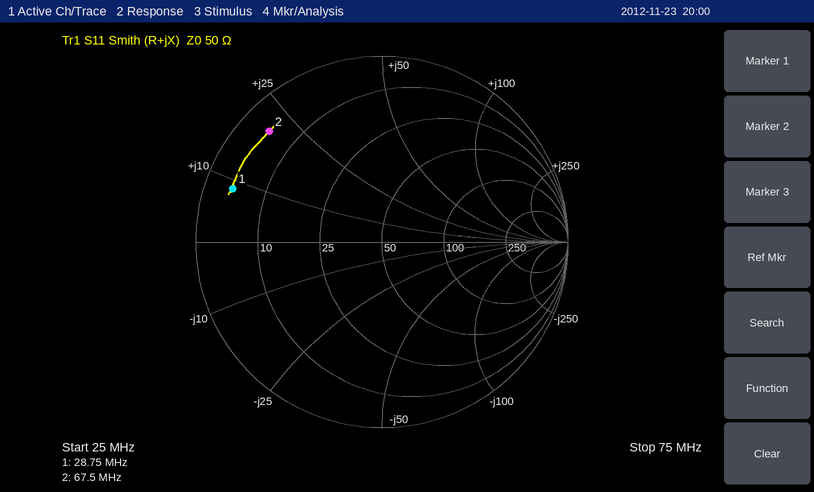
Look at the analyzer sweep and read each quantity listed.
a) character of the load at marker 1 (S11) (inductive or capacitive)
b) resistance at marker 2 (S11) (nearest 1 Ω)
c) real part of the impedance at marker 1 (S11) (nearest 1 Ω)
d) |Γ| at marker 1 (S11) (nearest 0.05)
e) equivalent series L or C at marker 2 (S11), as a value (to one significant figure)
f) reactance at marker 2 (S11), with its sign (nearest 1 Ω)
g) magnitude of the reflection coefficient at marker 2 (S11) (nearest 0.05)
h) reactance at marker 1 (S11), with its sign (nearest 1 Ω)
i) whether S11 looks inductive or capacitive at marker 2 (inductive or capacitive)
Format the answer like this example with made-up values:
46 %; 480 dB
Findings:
inductive; 5 Ω; 4 Ω; 0.85; 50 nH; +20 Ω; 0.85; +9 Ω; inductive
